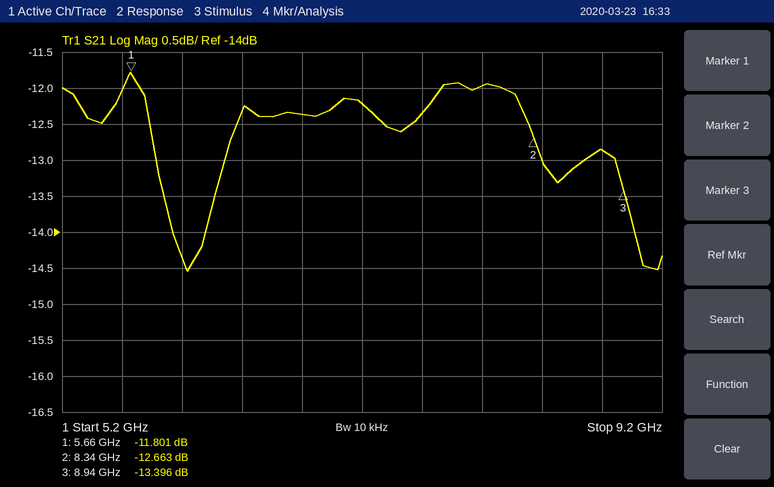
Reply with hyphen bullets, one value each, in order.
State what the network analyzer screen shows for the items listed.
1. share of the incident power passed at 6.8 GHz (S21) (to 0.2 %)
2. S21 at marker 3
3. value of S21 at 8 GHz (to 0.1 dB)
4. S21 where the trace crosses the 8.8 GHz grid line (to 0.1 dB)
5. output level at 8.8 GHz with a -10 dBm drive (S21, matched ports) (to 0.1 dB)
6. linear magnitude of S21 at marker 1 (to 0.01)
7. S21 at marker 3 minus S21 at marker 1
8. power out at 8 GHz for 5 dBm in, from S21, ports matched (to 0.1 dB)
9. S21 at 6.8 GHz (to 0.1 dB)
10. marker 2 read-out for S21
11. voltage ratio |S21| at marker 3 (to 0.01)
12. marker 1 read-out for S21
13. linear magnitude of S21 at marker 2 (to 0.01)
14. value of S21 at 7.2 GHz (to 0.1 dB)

- 5.8 %
- -13.396 dB
- -12.0 dB
- -12.9 dB
- -22.9 dBm
- 0.26
- -1.595 dB
- -7.0 dBm
- -12.4 dB
- -12.663 dB
- 0.21
- -11.801 dB
- 0.23
- -12.2 dB
